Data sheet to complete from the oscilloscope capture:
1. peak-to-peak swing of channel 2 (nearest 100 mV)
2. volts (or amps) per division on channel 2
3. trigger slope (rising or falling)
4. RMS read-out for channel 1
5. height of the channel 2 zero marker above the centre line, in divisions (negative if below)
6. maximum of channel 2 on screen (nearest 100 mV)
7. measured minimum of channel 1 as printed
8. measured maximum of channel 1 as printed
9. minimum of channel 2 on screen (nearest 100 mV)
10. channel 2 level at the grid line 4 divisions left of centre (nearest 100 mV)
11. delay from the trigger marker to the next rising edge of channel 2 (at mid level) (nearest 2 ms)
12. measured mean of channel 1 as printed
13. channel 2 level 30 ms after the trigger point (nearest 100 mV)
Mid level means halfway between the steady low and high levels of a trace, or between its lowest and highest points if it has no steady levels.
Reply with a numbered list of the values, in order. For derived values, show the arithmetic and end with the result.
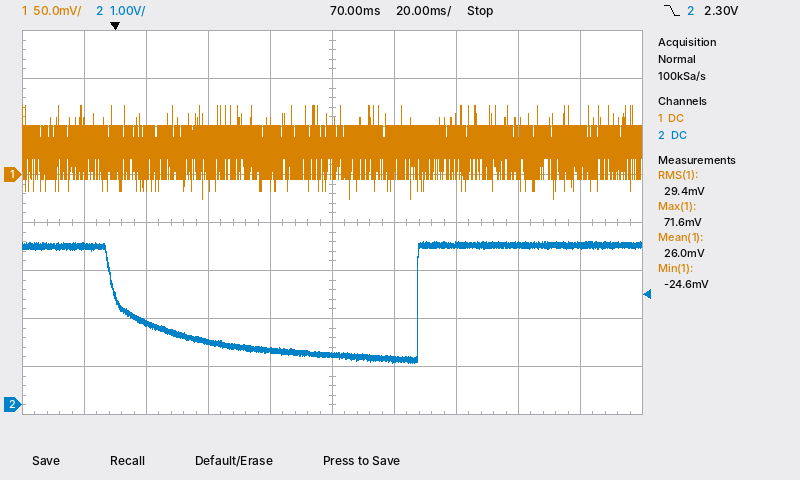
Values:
1. 3.4 V − (900 mV) = 2.5 V
2. 1 V
3. falling
4. 29.4 mV
5. -3.8 div
6. 3.4 V
7. -24.6 mV
8. 71.6 mV
9. 900 mV
10. 3.3 V
11. 98 ms
12. 26.0 mV
13. 1.3 V
